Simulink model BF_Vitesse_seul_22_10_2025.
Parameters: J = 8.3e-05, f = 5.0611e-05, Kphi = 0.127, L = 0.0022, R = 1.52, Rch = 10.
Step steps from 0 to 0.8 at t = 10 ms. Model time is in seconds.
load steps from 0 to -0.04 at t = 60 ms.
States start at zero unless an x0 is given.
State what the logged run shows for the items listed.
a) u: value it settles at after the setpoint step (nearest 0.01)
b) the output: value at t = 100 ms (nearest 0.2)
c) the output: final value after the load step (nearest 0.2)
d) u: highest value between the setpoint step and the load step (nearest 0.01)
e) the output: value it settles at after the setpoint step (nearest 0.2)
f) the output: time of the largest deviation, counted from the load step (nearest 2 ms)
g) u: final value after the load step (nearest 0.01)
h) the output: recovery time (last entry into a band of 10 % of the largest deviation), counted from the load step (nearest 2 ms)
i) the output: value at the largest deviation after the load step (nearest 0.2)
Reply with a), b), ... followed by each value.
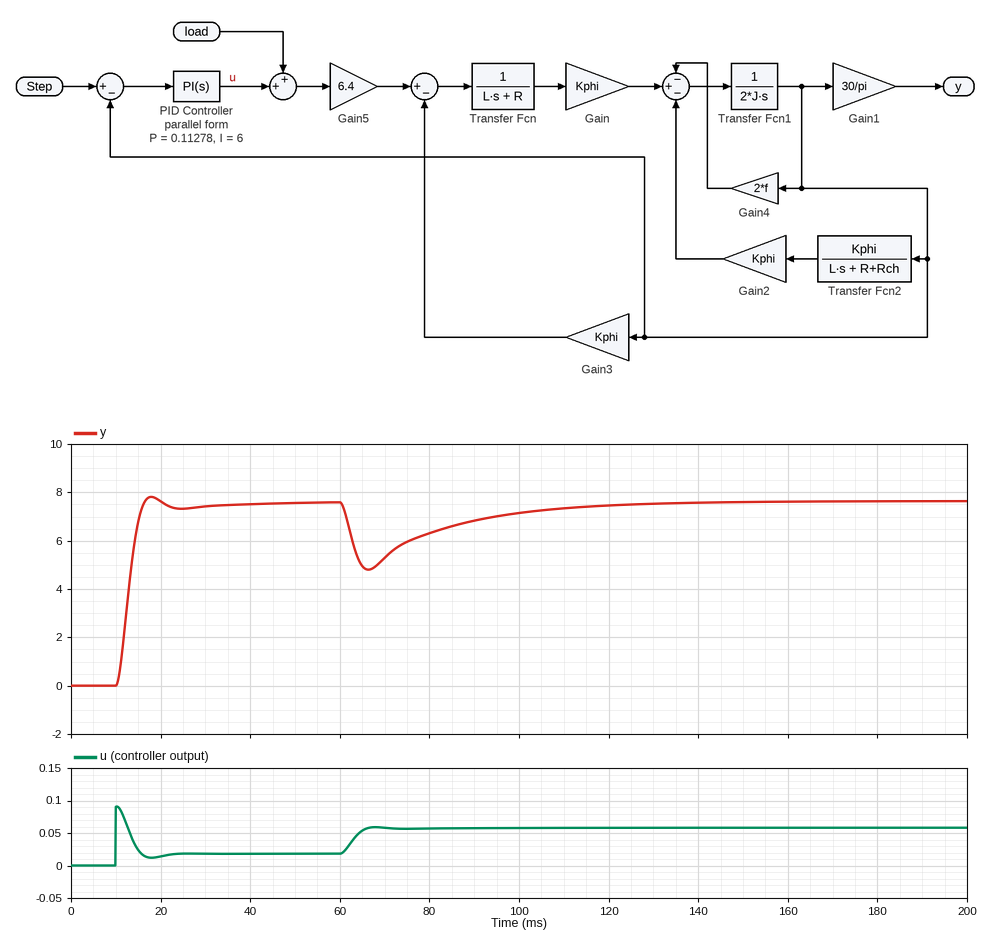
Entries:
a) 0.02
b) 7.2
c) 7.6
d) 0.09
e) 7.6
f) 6 ms
g) 0.06
h) 52 ms
i) 4.8
